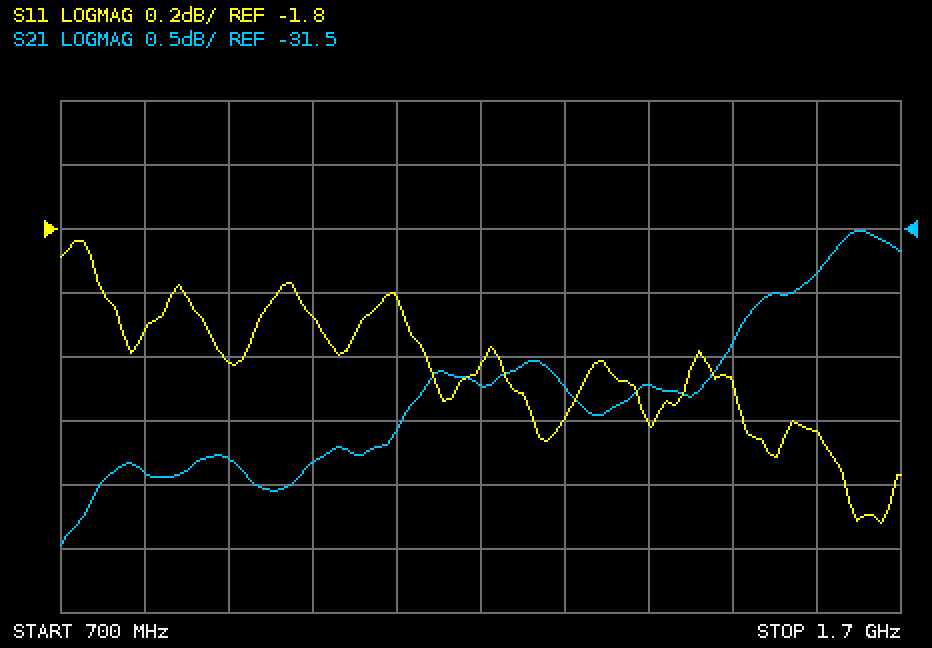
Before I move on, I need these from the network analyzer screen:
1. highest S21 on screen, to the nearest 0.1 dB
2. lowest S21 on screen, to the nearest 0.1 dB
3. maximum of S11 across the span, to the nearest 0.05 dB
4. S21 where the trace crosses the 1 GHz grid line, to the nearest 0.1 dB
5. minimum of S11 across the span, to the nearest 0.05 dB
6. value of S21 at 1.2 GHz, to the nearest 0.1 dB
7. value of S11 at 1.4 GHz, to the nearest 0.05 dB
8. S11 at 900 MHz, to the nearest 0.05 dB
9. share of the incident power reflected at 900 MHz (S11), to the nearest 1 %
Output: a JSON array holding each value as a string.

["-31.5 dB", "-34.0 dB", "-1.85 dB", "-33.3 dB", "-2.70 dB", "-32.7 dB", "-2.40 dB", "-2.20 dB", "60 %"]
